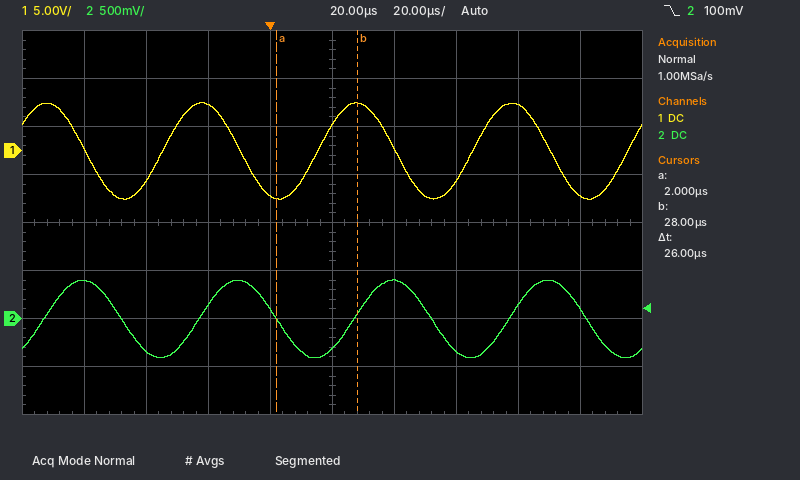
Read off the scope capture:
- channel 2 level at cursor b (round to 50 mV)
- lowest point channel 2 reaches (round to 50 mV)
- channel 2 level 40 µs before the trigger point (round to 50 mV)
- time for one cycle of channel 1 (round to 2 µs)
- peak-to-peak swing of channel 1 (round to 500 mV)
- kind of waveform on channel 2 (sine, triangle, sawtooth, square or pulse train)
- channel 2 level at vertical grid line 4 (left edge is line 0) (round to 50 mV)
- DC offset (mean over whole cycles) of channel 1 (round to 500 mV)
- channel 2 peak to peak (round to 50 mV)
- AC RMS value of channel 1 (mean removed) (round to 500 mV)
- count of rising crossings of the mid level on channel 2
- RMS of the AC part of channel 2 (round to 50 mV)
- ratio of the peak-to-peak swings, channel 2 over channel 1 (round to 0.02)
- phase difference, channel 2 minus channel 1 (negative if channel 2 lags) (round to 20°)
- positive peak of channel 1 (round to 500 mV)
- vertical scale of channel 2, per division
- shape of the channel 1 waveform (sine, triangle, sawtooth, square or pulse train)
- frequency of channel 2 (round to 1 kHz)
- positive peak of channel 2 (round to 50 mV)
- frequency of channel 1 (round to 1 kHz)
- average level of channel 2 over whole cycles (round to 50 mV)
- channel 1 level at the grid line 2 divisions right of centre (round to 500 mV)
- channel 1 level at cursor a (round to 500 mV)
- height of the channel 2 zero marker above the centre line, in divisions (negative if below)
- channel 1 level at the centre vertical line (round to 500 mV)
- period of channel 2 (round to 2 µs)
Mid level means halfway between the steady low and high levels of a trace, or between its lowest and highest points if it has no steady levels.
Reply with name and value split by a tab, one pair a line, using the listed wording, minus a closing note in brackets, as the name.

channel 2 level at cursor b	50 mV
lowest point channel 2 reaches	-400 mV
channel 2 level 40 µs before the trigger point	-350 mV
time for one cycle of channel 1	50 µs
peak-to-peak swing of channel 1	10.0 V
kind of waveform on channel 2	sine
channel 2 level at vertical grid line 4 (left edge is line 0)	100 mV
DC offset (mean over whole cycles) of channel 1	0.0 V
channel 2 peak to peak	800 mV
AC RMS value of channel 1 (mean removed)	3.5 V
count of rising crossings of the mid level on channel 2	4
RMS of the AC part of channel 2	300 mV
ratio of the peak-to-peak swings, channel 2 over channel 1	0.08
phase difference, channel 2 minus channel 1 (negative if channel 2 lags)	-80°
positive peak of channel 1	5.0 V
vertical scale of channel 2, per division	500 mV
shape of the channel 1 waveform	sine
frequency of channel 2	20 kHz
positive peak of channel 2	400 mV
frequency of channel 1	20 kHz
average level of channel 2 over whole cycles	0 mV
channel 1 level at the grid line 2 divisions right of centre	-3.0 V
channel 1 level at cursor a	-5.0 V
height of the channel 2 zero marker above the centre line, in divisions	-2.0 div
channel 1 level at the centre vertical line	2.5 V
period of channel 2	50 µs
